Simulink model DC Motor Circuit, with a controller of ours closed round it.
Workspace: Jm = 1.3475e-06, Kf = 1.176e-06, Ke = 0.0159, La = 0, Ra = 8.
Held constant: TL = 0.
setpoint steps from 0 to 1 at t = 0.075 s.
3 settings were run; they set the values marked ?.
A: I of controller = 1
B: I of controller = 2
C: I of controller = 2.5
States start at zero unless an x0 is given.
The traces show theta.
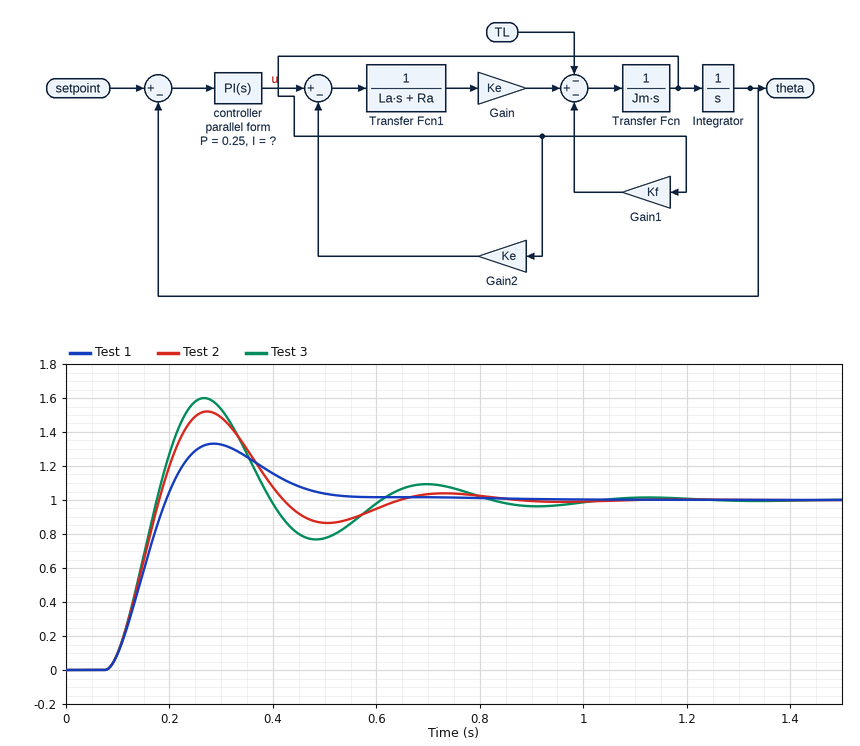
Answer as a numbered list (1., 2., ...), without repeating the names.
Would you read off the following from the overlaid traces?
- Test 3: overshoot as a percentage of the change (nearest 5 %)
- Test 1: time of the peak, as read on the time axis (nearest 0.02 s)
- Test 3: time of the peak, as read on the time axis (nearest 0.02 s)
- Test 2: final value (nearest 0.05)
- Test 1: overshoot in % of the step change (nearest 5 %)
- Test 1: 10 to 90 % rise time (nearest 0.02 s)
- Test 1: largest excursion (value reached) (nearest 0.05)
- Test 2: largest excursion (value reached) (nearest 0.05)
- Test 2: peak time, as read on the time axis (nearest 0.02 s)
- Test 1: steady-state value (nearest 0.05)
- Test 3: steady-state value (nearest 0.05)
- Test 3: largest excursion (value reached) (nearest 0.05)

1. 60 %
2. 0.28 s
3. 0.26 s
4. 1.00
5. 35 %
6. 0.08 s
7. 1.35
8. 1.50
9. 0.28 s
10. 1.00
11. 1.00
12. 1.60
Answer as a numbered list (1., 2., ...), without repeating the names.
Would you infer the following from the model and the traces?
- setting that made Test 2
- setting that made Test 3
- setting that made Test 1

1. B
2. C
3. A
